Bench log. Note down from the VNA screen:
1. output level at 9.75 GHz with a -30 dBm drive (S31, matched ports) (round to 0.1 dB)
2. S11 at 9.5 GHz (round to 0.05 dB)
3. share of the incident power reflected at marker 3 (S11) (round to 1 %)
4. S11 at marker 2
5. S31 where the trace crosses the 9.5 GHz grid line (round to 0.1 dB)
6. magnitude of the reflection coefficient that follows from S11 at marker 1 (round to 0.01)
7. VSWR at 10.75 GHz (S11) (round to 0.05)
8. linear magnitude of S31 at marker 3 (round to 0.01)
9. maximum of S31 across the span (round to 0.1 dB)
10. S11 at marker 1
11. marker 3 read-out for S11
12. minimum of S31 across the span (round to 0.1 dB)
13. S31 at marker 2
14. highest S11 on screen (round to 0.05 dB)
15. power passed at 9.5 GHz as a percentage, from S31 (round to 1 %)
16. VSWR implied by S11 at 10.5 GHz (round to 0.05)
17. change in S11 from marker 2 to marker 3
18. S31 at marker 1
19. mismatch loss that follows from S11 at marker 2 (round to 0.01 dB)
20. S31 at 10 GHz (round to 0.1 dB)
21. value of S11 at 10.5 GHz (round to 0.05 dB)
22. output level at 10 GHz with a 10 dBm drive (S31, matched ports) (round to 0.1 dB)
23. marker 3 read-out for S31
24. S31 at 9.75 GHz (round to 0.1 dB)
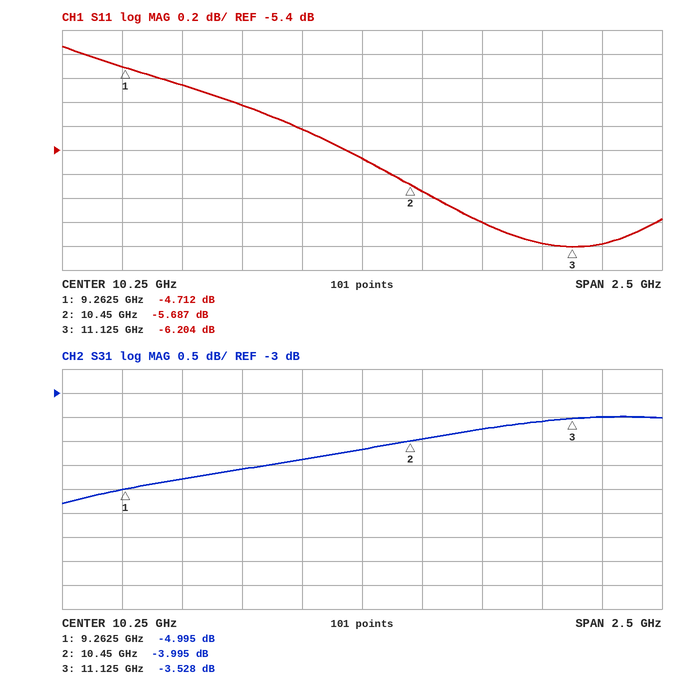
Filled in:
-34.6 dBm
-4.85 dB
24 %
-5.687 dB
-4.8 dB
0.58
3.00
0.67
-3.5 dB
-4.712 dB
-6.204 dB
-5.3 dB
-3.995 dB
-4.55 dB
33 %
3.15
-0.517 dB
-4.995 dB
1.37 dB
-4.4 dB
-5.75 dB
5.6 dBm
-3.528 dB
-4.6 dB
